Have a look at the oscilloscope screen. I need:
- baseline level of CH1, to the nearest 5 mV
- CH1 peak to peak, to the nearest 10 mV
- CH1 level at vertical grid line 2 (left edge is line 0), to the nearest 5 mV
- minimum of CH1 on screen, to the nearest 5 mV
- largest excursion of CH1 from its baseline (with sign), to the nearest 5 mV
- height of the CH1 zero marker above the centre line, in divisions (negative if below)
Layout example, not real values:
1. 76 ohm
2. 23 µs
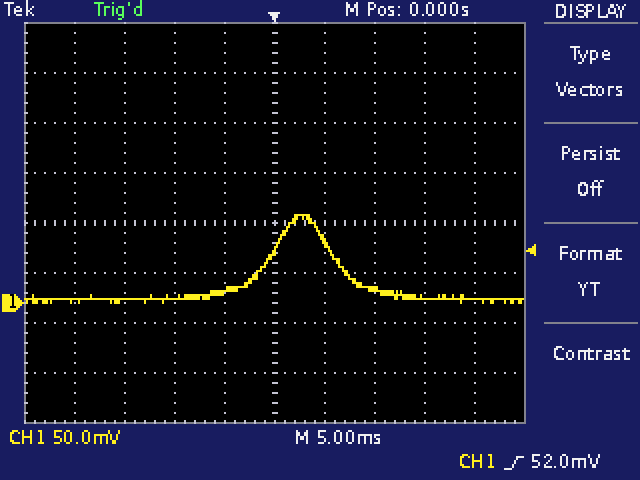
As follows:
1. 5 mV
2. 90 mV
3. 5 mV
4. 0 mV
5. +85 mV
6. -1.6 div
